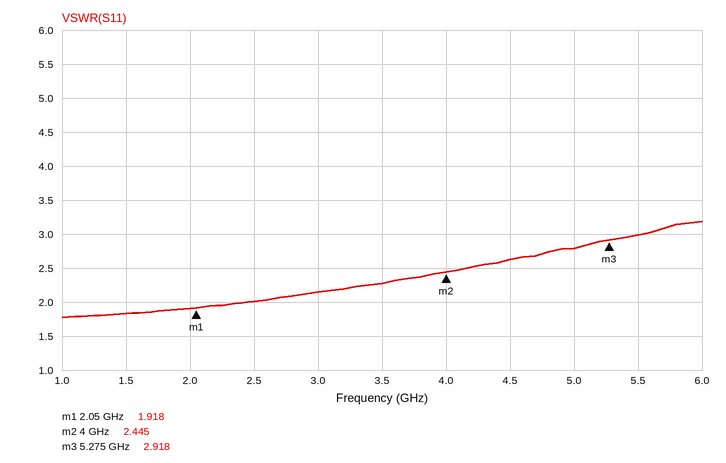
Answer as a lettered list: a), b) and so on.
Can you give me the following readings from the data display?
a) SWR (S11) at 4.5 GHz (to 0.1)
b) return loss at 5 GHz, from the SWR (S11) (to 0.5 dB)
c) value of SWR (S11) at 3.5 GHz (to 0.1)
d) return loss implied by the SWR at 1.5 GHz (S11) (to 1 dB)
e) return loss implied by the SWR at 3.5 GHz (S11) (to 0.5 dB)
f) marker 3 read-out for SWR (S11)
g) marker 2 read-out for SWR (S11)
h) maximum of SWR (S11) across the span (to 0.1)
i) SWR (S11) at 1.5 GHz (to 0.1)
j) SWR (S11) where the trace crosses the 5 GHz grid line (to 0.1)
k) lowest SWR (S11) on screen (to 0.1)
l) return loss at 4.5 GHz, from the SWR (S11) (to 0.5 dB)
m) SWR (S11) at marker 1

a) 2.6
b) 6.5 dB
c) 2.3
d) 11 dB
e) 8.0 dB
f) 2.918
g) 2.445
h) 3.2
i) 1.8
j) 2.8
k) 1.8
l) 7.0 dB
m) 1.918
